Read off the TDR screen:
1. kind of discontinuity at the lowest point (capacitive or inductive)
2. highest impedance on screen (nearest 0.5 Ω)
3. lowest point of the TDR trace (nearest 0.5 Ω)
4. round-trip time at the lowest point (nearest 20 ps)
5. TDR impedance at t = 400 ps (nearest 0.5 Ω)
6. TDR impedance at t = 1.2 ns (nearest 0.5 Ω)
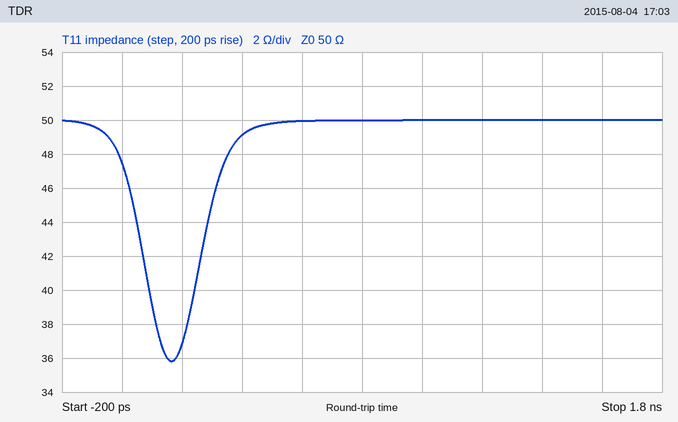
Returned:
capacitive
50.0 Ω
36.0 Ω
160 ps
49.0 Ω
50.0 Ω
